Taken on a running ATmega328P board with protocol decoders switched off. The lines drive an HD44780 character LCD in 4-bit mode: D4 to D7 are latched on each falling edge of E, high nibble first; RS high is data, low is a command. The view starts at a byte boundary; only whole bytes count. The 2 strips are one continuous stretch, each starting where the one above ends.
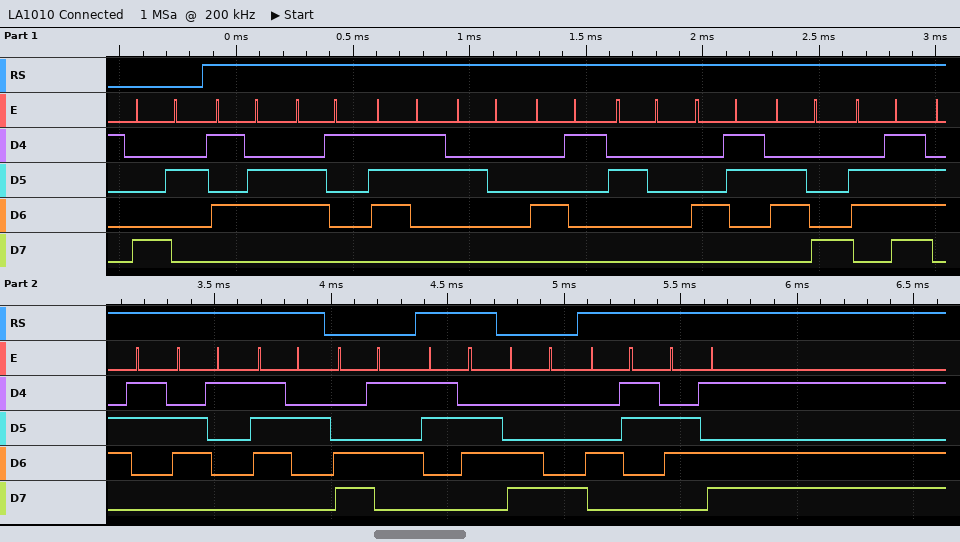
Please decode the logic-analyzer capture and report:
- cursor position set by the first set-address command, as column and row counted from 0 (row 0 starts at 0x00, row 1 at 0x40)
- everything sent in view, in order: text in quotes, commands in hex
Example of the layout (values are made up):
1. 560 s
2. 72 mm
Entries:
1. column 2, row 0
2. 0x82 "Vas A Chocar" 0xC5 "6" 0xC8 "Cm"
